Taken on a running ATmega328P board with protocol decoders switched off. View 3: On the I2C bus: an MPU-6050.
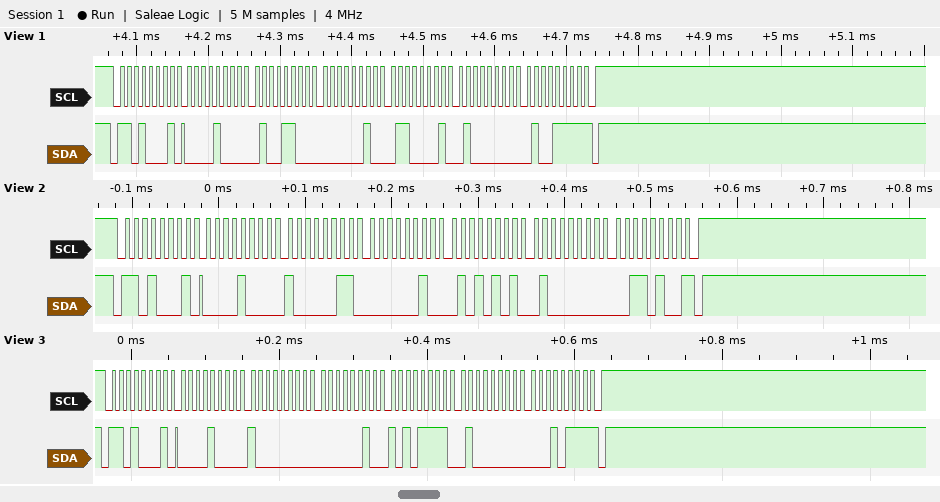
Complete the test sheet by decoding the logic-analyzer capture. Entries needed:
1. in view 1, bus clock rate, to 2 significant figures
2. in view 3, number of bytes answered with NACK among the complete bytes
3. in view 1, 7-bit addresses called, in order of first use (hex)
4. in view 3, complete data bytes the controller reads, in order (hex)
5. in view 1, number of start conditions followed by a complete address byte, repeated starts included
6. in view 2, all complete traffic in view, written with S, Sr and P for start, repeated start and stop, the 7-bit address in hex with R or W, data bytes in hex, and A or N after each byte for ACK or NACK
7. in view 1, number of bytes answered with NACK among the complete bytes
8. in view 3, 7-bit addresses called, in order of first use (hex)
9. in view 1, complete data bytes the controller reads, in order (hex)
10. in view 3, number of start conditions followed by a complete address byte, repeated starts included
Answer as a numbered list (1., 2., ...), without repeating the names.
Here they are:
1. 100 kHz
2. 1
3. 0x68
4. 08 80 02 AF 40 17
5. 1
6. S 68R A 08 A 83 A 02 A 55 A 40 A 34 N P
7. 1
8. 0x68
9. 08 4C 02 61 40 4F
10. 1
